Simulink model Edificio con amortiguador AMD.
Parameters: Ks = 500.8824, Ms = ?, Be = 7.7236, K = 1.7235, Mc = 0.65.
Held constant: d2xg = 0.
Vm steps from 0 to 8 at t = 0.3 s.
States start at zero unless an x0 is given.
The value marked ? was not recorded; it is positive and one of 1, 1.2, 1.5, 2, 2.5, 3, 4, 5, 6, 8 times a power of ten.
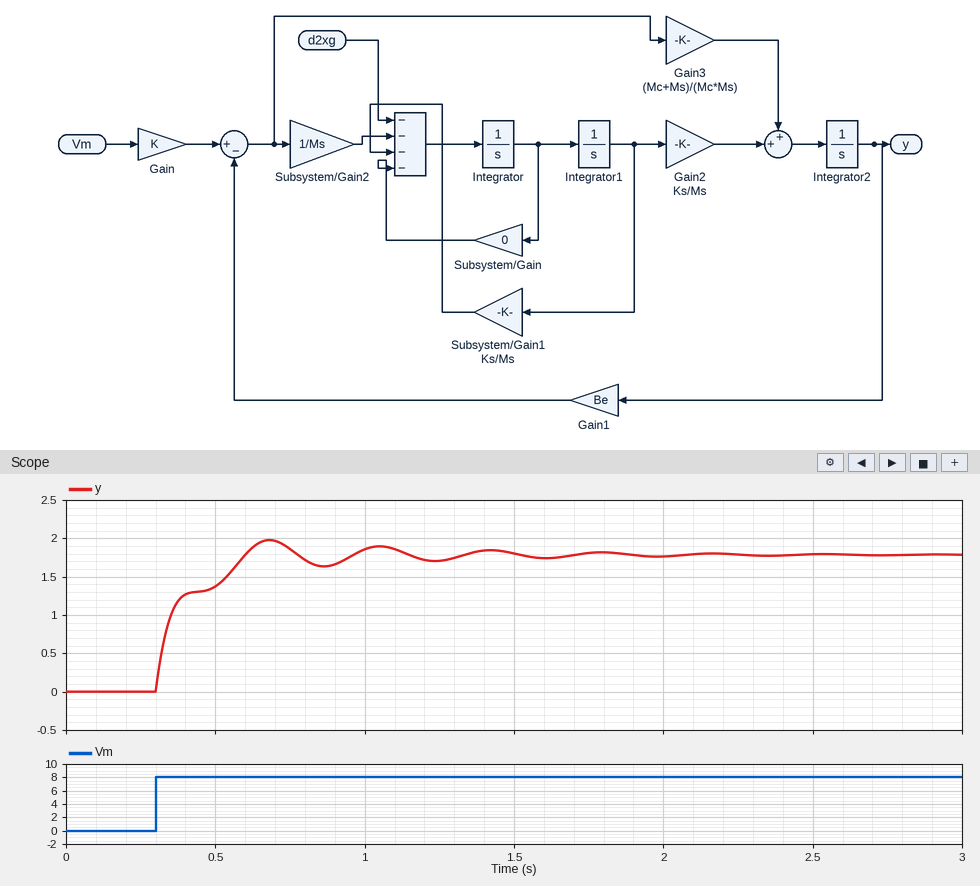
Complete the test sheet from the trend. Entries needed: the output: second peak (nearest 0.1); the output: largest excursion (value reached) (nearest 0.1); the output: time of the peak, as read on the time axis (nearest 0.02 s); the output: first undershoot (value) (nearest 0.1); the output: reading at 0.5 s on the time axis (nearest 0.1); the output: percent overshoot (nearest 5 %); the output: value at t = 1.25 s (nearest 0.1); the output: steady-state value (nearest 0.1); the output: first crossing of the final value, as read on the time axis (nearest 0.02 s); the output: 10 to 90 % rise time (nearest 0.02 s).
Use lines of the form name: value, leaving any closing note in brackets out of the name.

the output: second peak: 1.9
the output: largest excursion (value reached): 2.0
the output: time of the peak, as read on the time axis: 0.68 s
the output: first undershoot (value): 1.6
the output: reading at 0.5 s on the time axis: 1.4
the output: percent overshoot: 10 %
the output: value at t = 1.25 s: 1.7
the output: steady-state value: 1.8
the output: first crossing of the final value, as read on the time axis: 0.60 s
the output: 10 to 90 % rise time: 0.26 s
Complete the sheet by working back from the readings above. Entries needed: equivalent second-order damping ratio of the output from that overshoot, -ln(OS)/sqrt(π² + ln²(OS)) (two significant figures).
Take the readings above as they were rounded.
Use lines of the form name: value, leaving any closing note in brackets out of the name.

equivalent second-order damping ratio of the output from that overshoot, -ln(OS)/sqrt(π² + ln²(OS)): 0.59
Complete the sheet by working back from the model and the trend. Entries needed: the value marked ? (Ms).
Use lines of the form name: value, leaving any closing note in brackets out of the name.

the value marked ?: 1.5
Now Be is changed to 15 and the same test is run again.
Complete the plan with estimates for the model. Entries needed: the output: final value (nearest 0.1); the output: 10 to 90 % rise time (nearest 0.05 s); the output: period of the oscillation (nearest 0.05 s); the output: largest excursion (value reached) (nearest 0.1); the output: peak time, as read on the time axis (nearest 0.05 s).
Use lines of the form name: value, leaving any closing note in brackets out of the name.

the output: final value: 0.9
the output: 10 to 90 % rise time: 0.20 s
the output: period of the oscillation: 0.40 s
the output: largest excursion (value reached): 1.0
the output: peak time, as read on the time axis: 0.65 s
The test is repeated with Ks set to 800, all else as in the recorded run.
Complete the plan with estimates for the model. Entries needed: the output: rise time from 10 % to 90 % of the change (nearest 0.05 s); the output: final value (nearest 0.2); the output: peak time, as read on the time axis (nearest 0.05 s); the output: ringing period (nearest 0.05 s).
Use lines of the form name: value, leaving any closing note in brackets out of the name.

the output: rise time from 10 % to 90 % of the change: 0.20 s
the output: final value: 1.8
the output: peak time, as read on the time axis: 0.60 s
the output: ringing period: 0.30 s
